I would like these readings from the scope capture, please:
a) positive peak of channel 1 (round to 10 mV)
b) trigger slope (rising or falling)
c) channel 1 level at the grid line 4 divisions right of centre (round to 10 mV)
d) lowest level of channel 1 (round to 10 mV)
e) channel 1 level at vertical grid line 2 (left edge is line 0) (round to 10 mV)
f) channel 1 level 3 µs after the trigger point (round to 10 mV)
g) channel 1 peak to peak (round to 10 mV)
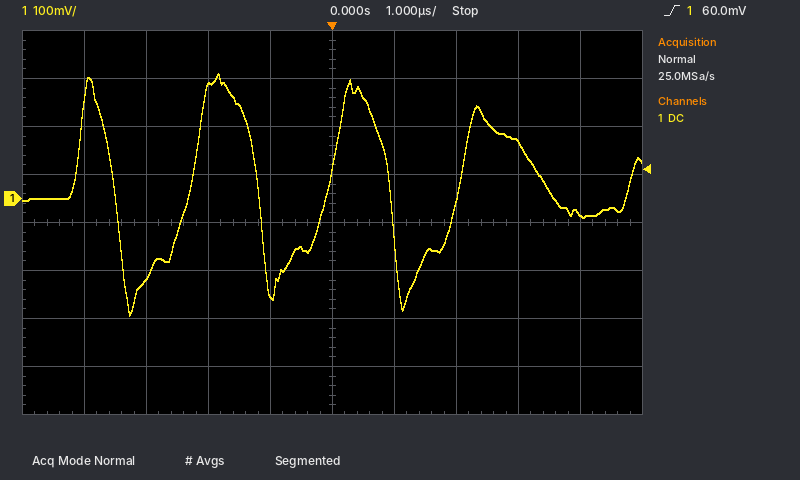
260 mV
rising
-30 mV
-240 mV
-170 mV
120 mV
500 mV
